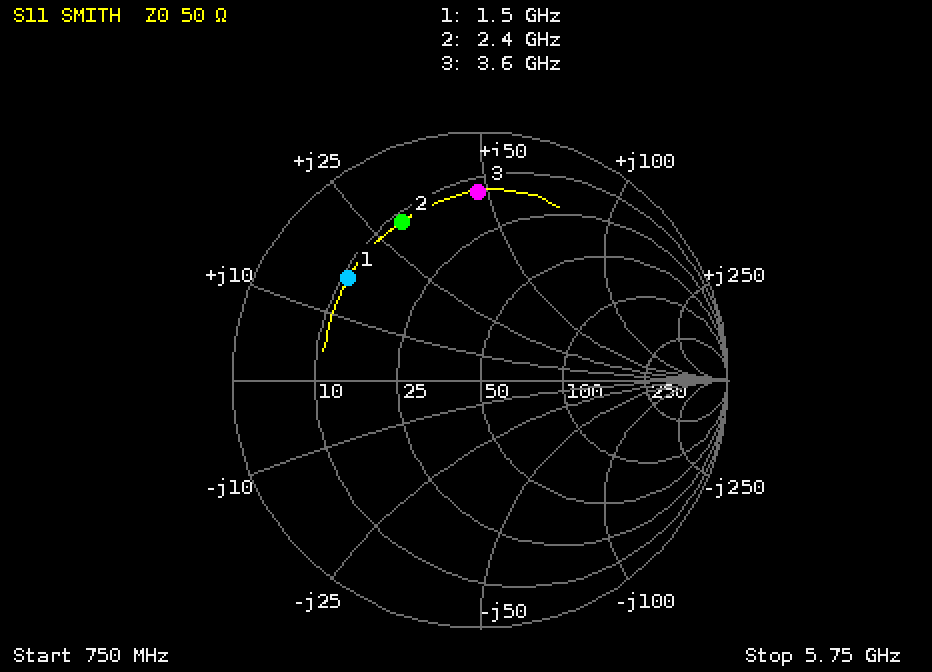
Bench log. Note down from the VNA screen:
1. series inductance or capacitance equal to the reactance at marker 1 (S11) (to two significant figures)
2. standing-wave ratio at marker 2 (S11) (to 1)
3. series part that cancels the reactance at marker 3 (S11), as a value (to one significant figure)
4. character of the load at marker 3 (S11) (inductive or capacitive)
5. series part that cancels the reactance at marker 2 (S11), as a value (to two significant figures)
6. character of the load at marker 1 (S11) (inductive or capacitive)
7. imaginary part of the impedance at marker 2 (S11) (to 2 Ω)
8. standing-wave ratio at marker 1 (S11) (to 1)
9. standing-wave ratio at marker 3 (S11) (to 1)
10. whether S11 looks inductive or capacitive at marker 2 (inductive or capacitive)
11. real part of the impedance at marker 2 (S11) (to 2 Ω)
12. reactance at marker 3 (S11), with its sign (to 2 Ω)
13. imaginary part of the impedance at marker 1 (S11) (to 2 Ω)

1.7 nH
6
900 fF
inductive
2.2 pF
inductive
+30 Ω
5
7
inductive
12 Ω
+48 Ω
+16 Ω
